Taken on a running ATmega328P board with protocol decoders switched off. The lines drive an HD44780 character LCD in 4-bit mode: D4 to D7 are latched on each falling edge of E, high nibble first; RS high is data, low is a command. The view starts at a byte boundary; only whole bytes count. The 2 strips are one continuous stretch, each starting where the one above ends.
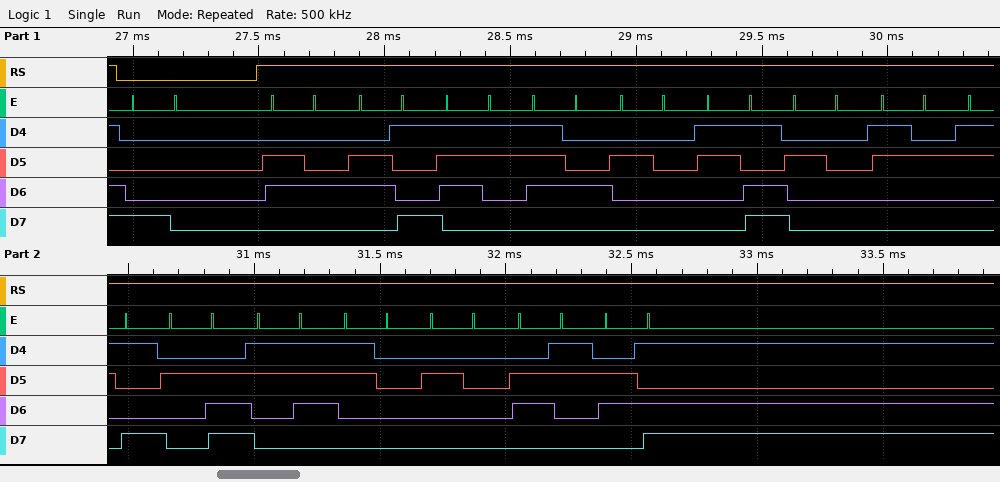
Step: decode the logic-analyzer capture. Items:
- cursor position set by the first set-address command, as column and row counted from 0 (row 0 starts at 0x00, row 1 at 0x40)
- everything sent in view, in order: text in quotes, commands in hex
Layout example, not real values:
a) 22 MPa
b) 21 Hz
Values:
a) column 0, row 0
b) 0x80 "dist = 29.70 cm"
